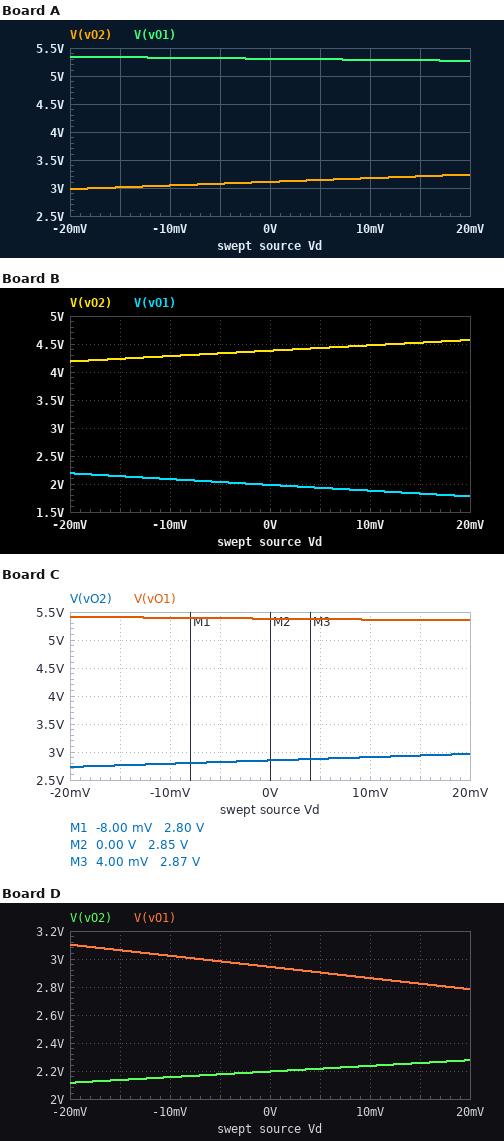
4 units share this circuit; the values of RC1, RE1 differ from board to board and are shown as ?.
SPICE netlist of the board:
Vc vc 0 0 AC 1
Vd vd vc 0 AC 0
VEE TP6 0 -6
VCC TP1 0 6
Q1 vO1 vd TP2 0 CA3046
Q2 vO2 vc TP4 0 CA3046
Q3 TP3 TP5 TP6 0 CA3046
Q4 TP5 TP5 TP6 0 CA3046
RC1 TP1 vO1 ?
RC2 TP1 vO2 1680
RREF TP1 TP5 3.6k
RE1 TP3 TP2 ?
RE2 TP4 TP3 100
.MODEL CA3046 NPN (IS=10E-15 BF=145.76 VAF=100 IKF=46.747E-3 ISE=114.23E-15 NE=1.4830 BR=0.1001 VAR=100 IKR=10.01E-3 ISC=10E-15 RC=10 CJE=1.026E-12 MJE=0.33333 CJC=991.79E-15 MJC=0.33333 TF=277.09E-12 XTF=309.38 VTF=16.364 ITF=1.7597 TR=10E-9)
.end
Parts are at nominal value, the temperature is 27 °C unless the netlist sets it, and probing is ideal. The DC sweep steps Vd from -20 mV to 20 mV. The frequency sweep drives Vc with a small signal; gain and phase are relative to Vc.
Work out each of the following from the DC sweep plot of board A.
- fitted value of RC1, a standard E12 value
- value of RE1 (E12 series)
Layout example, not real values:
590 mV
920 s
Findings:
470 Ω
120 Ω
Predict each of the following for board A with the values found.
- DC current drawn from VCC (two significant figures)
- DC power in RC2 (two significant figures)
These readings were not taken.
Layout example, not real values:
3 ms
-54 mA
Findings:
6.3 mA
5.0 mW
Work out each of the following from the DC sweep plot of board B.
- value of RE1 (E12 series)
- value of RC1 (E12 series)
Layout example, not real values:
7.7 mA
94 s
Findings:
33 Ω
1.8 kΩ
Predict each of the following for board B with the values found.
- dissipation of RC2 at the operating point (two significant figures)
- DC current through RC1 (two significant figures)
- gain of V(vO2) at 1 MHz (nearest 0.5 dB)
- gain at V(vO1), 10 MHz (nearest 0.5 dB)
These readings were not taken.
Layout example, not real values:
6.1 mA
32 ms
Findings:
1.6 mW
2.2 mA
-37.0 dB
-27.0 dB
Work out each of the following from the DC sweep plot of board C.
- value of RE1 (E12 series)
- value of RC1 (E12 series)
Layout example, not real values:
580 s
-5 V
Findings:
150 Ω
470 Ω
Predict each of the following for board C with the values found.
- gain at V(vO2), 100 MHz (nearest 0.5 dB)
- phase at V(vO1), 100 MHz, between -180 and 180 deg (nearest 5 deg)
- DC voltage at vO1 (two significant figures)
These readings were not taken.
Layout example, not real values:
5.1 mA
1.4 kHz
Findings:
-12.5 dB
130 deg
5.4 V
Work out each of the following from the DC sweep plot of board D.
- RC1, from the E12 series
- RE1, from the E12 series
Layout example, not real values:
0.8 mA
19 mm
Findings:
3.3 kΩ
270 Ω
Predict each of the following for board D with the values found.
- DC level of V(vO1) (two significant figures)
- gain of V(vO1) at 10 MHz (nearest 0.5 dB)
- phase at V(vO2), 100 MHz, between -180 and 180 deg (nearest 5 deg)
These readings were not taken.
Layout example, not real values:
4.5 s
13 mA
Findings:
2.9 V
-23.0 dB
145 deg
